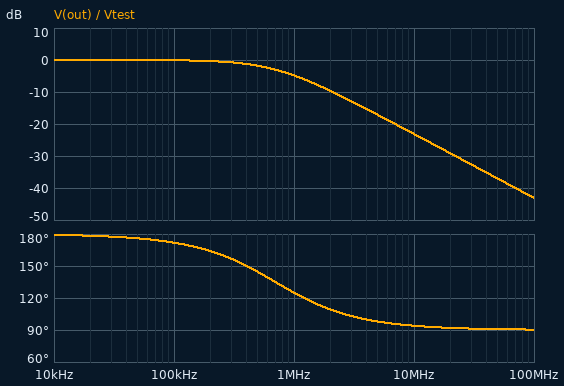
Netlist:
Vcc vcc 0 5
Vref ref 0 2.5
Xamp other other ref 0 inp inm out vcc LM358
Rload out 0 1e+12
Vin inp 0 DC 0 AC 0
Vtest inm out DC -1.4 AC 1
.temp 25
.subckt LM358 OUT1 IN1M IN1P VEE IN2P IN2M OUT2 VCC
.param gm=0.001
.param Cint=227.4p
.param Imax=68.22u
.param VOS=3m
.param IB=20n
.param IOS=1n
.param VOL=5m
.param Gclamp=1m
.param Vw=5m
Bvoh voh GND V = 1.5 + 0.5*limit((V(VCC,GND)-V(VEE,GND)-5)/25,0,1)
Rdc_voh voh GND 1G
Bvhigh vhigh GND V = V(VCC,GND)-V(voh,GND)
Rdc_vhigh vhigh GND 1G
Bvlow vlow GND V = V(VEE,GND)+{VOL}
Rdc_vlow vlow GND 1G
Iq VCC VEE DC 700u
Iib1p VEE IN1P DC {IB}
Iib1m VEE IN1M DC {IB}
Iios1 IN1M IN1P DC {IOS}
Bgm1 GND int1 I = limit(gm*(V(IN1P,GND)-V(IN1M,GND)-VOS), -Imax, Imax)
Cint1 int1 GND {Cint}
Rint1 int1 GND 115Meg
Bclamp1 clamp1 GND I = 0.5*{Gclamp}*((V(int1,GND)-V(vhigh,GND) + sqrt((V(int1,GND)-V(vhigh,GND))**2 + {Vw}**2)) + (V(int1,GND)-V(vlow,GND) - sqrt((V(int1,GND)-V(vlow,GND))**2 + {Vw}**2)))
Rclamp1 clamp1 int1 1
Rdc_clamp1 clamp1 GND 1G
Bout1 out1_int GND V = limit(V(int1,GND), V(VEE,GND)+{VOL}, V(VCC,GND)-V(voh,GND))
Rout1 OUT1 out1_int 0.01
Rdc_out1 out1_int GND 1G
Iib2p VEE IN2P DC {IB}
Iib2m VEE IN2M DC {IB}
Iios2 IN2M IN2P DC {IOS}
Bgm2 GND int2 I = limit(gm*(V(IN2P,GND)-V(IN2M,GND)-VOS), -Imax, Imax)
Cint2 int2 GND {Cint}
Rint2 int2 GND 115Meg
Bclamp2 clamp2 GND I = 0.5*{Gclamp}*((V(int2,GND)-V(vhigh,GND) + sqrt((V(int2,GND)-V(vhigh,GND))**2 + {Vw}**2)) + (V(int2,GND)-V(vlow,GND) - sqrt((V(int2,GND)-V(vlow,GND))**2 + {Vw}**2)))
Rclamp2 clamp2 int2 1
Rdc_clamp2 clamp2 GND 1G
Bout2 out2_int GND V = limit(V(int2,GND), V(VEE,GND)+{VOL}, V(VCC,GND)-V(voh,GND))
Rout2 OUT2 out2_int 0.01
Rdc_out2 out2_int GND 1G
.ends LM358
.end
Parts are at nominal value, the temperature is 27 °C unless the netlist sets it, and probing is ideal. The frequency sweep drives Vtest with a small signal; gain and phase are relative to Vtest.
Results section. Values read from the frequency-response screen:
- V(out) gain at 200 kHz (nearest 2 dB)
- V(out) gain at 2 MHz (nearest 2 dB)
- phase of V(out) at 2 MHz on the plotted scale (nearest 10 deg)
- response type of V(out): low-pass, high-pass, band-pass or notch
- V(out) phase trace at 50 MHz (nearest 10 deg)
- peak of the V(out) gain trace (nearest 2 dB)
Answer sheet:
0 dB
-10 dB
110 deg
low-pass
90 deg
0 dB
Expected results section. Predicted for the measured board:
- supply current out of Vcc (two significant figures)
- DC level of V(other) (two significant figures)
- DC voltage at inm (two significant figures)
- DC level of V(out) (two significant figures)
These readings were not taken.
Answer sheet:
700 µA
2.5 V
-3.0 mV
1.4 V
